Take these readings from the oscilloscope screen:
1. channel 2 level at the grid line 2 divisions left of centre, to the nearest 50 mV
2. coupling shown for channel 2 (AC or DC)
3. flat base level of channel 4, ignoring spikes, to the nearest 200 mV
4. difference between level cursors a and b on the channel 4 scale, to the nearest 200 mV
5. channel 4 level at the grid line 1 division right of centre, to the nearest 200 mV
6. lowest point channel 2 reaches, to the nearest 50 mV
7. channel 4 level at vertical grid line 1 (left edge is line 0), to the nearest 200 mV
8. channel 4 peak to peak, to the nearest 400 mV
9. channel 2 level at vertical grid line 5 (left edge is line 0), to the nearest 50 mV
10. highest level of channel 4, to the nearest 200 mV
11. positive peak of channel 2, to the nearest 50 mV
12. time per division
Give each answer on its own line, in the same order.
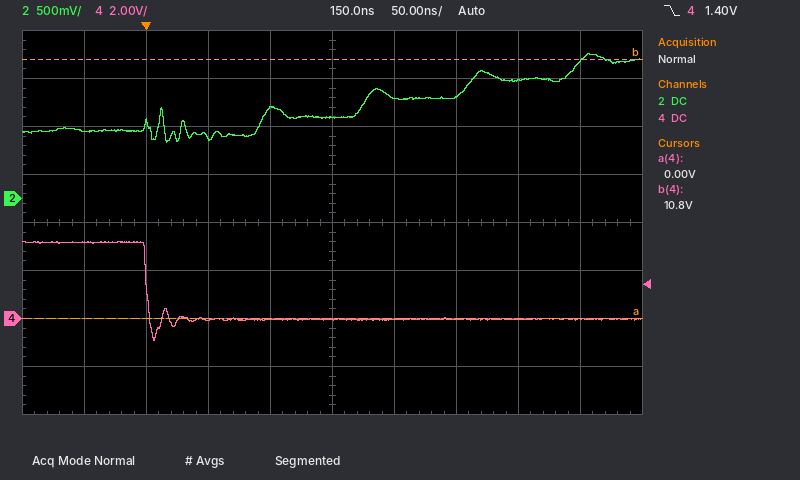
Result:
650 mV
DC
0.0 V
10.8 V
0.0 V
600 mV
3.2 V
4.0 V
850 mV
3.2 V
1.50 V
50 ns
